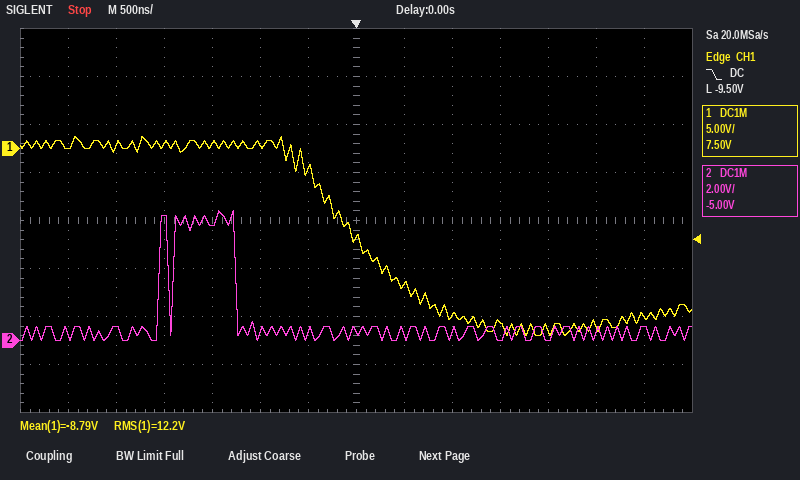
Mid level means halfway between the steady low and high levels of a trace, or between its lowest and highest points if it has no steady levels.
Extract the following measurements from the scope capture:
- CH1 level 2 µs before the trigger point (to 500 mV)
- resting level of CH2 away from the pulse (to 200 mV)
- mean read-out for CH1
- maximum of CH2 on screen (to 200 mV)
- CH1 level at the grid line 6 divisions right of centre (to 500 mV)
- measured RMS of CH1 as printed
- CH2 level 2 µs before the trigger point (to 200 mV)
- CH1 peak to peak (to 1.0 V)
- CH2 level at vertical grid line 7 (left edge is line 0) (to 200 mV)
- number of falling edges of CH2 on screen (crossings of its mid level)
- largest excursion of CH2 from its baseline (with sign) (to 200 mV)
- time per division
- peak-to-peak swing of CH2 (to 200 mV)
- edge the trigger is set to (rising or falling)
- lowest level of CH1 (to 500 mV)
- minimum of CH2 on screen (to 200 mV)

500 mV
400 mV
-8.79 V
5.4 V
-17.5 V
12.2 V
5.2 V
21.0 V
400 mV
2
+5.0 V
500 ns
5.4 V
falling
-19.5 V
0.0 V
